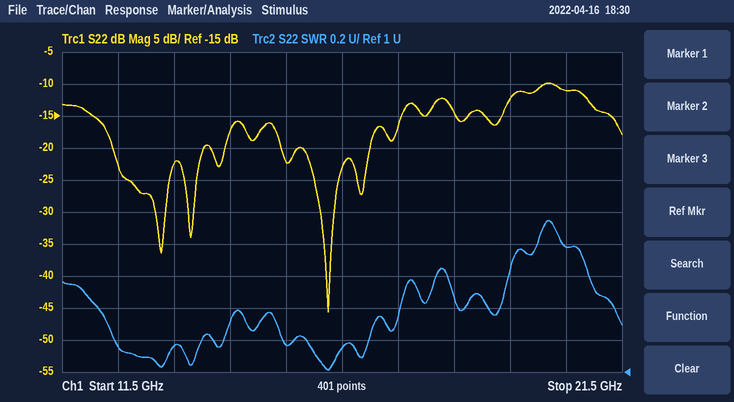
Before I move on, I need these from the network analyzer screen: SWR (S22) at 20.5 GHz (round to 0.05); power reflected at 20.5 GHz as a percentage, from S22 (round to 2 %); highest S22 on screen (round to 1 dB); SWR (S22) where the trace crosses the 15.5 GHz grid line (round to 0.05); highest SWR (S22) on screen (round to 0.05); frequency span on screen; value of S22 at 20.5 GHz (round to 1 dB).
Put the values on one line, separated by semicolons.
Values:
1.80; 8 %; -10 dB; 1.15; 1.95; 10 GHz; -11 dB
